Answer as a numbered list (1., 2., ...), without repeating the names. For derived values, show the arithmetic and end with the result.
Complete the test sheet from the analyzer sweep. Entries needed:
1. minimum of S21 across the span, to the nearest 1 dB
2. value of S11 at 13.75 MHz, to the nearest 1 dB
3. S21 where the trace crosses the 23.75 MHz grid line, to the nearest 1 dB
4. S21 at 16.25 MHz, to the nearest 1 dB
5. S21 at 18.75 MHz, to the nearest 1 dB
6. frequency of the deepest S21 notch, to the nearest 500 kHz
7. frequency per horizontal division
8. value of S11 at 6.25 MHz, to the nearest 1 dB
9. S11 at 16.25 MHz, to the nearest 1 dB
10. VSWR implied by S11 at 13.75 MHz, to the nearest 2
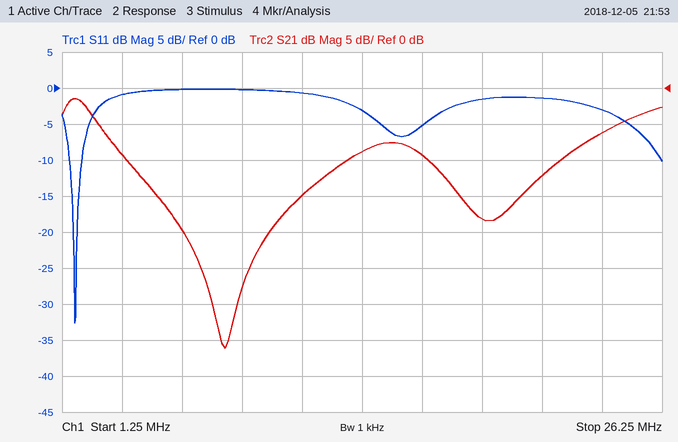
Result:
1. -36 dB
2. -3 dB
3. -6 dB
4. -9 dB
5. -18 dB
6. 8.0 MHz
7. 2.5 MHz
8. 0 dB
9. -5 dB
10. |Γ| = 10^(-3/20) = 0.7079; VSWR = (1 + 0.7079)/(1 − 0.7079) ≈ 6
